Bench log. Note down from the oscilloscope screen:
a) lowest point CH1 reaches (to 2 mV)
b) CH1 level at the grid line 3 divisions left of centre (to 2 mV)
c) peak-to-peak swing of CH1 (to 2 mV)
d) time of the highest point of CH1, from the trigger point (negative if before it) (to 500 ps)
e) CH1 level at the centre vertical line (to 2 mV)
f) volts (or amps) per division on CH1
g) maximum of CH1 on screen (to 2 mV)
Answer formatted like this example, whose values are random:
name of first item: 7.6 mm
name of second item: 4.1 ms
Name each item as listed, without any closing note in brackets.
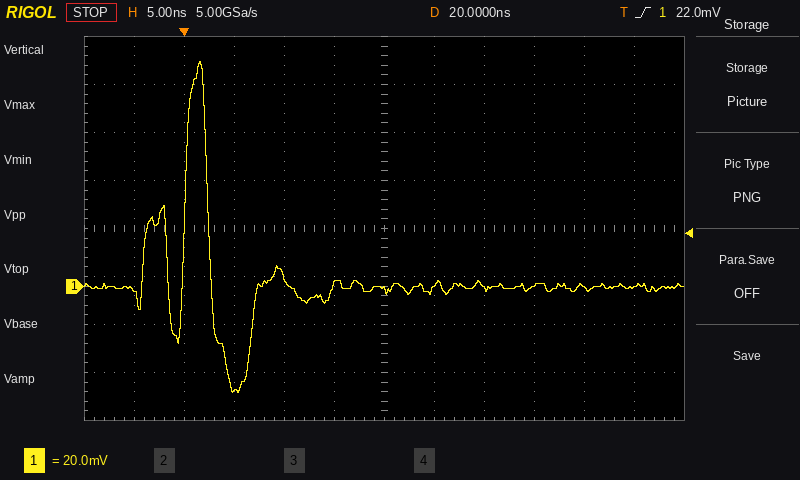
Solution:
lowest point CH1 reaches: -44 mV
CH1 level at the grid line 3 divisions left of centre: -44 mV
peak-to-peak swing of CH1: 138 mV
time of the highest point of CH1, from the trigger point (negative if before it): +1.5 ns
CH1 level at the centre vertical line: -2 mV
volts (or amps) per division on CH1: 20 mV
maximum of CH1 on screen: 94 mV
